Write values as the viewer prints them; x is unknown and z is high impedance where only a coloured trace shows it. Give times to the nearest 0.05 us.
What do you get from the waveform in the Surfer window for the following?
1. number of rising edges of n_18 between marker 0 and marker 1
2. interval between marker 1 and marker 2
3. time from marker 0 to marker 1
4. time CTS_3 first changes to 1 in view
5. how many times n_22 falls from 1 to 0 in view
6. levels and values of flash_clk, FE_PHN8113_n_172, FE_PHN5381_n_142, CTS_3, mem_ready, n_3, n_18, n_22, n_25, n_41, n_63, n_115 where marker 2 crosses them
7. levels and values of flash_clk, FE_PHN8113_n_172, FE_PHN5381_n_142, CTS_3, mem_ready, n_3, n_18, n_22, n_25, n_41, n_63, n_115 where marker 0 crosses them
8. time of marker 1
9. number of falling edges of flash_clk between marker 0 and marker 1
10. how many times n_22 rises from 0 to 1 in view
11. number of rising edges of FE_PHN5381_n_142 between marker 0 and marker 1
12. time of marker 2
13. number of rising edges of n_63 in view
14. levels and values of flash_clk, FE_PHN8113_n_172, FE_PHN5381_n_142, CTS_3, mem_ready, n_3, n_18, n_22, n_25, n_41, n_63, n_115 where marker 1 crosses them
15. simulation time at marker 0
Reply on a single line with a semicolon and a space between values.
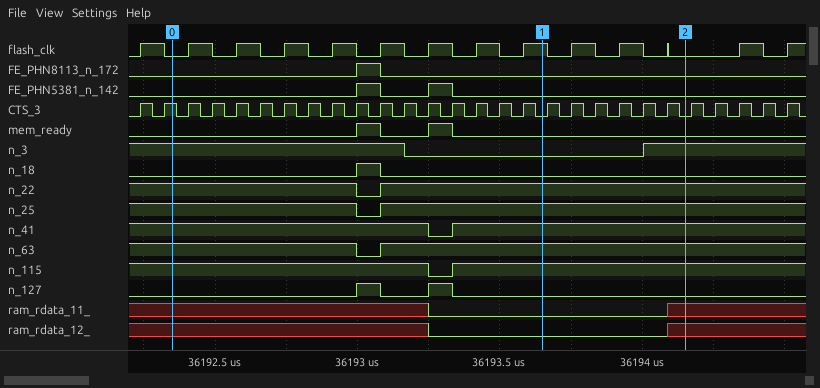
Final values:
1; 0.5 us; 1.3 us; 36192.25 us; 1; flash_clk=0, FE_PHN8113_n_172=0, FE_PHN5381_n_142=0, CTS_3=0, mem_ready=0, n_3=1, n_18=0, n_22=1, n_25=1, n_41=1, n_63=1, n_115=1; flash_clk=0, FE_PHN8113_n_172=0, FE_PHN5381_n_142=0, CTS_3=1, mem_ready=0, n_3=1, n_18=0, n_22=1, n_25=1, n_41=1, n_63=1, n_115=1; 36193.65 us; 7; 1; 2; 36194.15 us; 1; flash_clk=1, FE_PHN8113_n_172=0, FE_PHN5381_n_142=0, CTS_3=0, mem_ready=0, n_3=0, n_18=0, n_22=1, n_25=1, n_41=1, n_63=1, n_115=1; 36192.35 us
